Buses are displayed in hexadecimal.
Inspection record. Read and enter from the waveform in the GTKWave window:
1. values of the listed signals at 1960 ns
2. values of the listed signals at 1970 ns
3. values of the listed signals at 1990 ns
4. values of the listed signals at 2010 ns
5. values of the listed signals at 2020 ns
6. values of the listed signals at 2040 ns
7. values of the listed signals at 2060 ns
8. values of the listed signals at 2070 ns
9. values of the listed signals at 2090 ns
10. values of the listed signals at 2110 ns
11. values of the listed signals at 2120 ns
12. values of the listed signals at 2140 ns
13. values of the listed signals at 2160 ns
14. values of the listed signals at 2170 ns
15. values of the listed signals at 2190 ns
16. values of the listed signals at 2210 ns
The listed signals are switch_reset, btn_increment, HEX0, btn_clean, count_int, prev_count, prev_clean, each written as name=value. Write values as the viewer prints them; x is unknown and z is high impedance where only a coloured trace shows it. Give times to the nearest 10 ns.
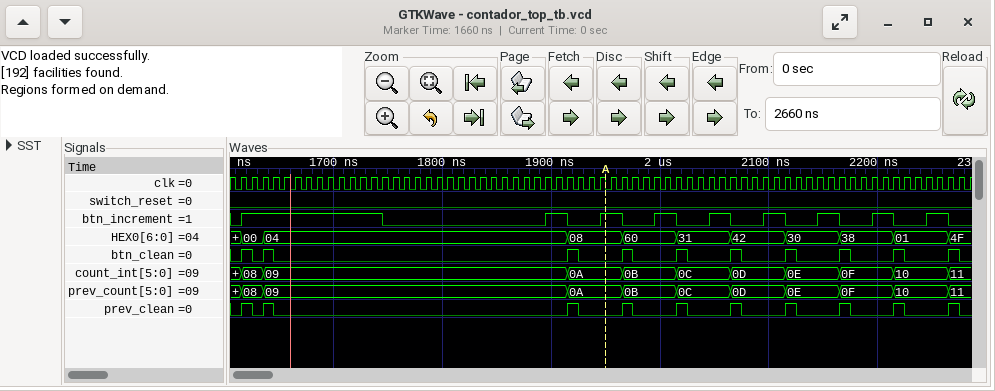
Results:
switch_reset=0, btn_increment=1, HEX0=08, btn_clean=0, count_int=0A, prev_count=0A, prev_clean=0
switch_reset=0, btn_increment=0, HEX0=60, btn_clean=1, count_int=0B, prev_count=0B, prev_clean=1
switch_reset=0, btn_increment=0, HEX0=60, btn_clean=0, count_int=0B, prev_count=0B, prev_clean=0
switch_reset=0, btn_increment=1, HEX0=60, btn_clean=0, count_int=0B, prev_count=0B, prev_clean=0
switch_reset=0, btn_increment=0, HEX0=31, btn_clean=1, count_int=0C, prev_count=0C, prev_clean=1
switch_reset=0, btn_increment=0, HEX0=31, btn_clean=0, count_int=0C, prev_count=0C, prev_clean=0
switch_reset=0, btn_increment=1, HEX0=31, btn_clean=0, count_int=0C, prev_count=0C, prev_clean=0
switch_reset=0, btn_increment=0, HEX0=42, btn_clean=1, count_int=0D, prev_count=0D, prev_clean=1
switch_reset=0, btn_increment=0, HEX0=42, btn_clean=0, count_int=0D, prev_count=0D, prev_clean=0
switch_reset=0, btn_increment=1, HEX0=42, btn_clean=0, count_int=0D, prev_count=0D, prev_clean=0
switch_reset=0, btn_increment=0, HEX0=30, btn_clean=1, count_int=0E, prev_count=0E, prev_clean=1
switch_reset=0, btn_increment=0, HEX0=30, btn_clean=0, count_int=0E, prev_count=0E, prev_clean=0
switch_reset=0, btn_increment=1, HEX0=30, btn_clean=0, count_int=0E, prev_count=0E, prev_clean=0
switch_reset=0, btn_increment=0, HEX0=38, btn_clean=1, count_int=0F, prev_count=0F, prev_clean=1
switch_reset=0, btn_increment=0, HEX0=38, btn_clean=0, count_int=0F, prev_count=0F, prev_clean=0
switch_reset=0, btn_increment=1, HEX0=38, btn_clean=0, count_int=0F, prev_count=0F, prev_clean=0
